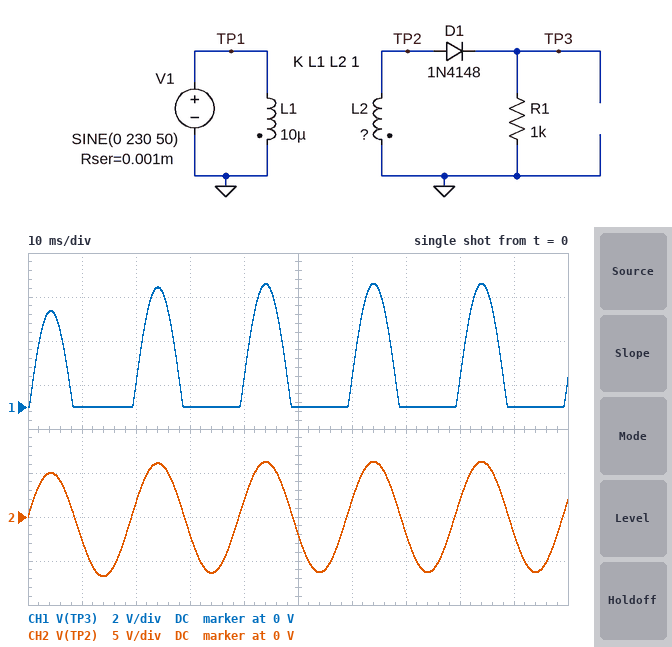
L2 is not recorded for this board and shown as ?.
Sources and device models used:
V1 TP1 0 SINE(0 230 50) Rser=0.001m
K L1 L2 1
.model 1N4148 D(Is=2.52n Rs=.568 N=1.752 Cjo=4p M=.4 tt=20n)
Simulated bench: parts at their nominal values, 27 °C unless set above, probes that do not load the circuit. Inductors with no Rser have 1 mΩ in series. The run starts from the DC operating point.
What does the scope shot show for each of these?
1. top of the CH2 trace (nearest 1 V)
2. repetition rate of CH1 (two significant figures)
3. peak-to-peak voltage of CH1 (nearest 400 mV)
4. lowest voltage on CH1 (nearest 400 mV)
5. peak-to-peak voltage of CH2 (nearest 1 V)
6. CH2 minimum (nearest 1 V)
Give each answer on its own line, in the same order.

6 V
51 Hz
5.6 V
0 V
13 V
-7 V
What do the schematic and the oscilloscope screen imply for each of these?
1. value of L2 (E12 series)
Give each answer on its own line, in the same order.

8.2 nH
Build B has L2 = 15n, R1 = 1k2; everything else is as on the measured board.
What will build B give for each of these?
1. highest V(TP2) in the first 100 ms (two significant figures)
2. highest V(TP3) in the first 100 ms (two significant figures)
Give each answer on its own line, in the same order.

8.5 V
7.8 V
